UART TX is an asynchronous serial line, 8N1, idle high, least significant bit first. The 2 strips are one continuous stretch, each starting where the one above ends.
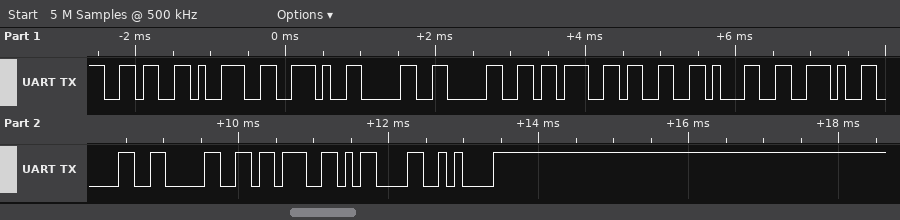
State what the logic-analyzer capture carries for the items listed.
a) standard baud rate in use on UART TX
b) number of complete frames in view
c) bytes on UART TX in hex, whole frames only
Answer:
9600 baud
14
0x36 0x39 0x2E 0x30 0x30 0x3B 0x33 0x31 0x2E 0x30 0x30 0x3B 0x0D 0x0A
